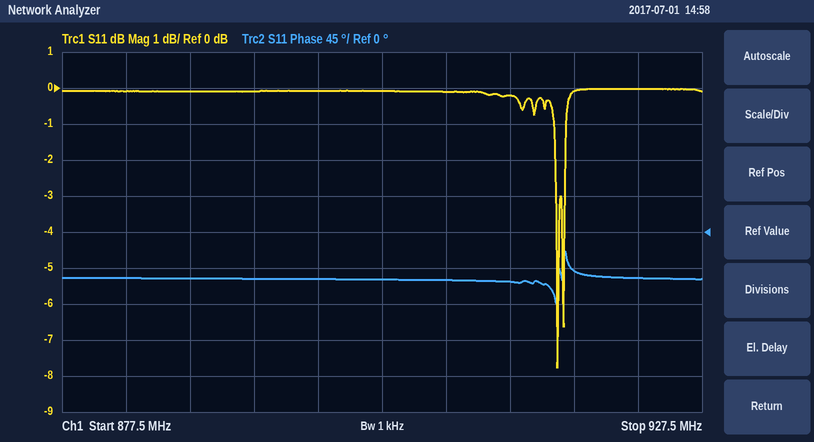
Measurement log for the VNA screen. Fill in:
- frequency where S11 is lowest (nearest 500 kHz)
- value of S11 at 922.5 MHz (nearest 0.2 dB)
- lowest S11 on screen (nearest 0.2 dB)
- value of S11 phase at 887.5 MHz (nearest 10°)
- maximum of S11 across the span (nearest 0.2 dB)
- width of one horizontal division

916.0 MHz
0.0 dB
-7.8 dB
-60°
0.0 dB
5 MHz
